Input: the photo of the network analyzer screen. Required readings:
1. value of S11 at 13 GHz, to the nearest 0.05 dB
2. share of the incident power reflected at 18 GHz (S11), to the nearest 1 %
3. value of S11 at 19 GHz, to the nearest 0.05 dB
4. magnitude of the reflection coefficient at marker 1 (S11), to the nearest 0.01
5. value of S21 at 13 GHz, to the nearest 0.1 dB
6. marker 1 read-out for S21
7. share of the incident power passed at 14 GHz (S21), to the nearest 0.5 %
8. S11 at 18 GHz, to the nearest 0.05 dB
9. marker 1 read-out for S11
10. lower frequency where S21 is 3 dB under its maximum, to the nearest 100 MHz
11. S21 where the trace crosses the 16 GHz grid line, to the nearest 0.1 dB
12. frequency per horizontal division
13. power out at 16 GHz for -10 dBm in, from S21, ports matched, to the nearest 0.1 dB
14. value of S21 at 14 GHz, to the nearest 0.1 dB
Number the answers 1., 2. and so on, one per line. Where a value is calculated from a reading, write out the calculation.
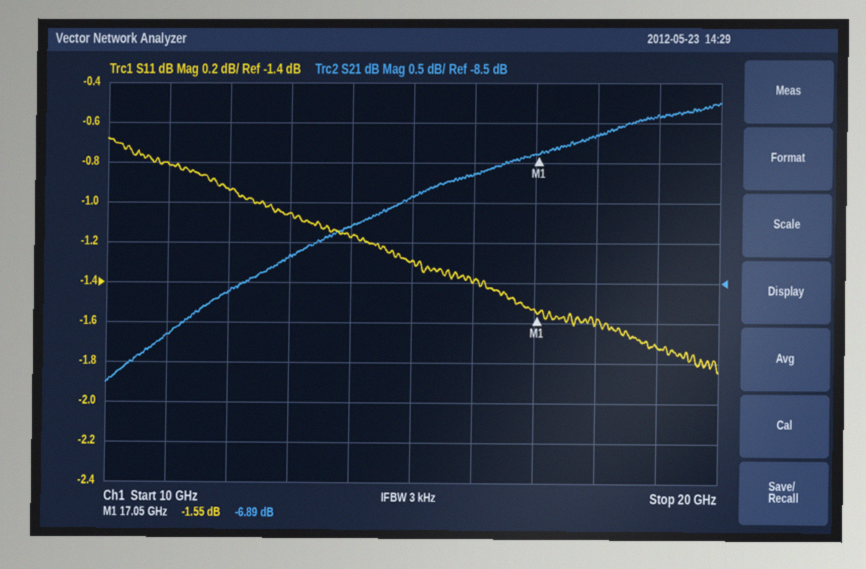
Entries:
1. -1.05 dB
2. 10^(-1.6/10) ≈ 69 %
3. -1.70 dB
4. 10^(-1.55/20) ≈ 0.84
5. -8.2 dB
6. -6.89 dB
7. 10^(-7.8/10) ≈ 16.6 %, so 16.5 % to the nearest 0.5 %
8. -1.60 dB
9. -1.55 dB
10. 10.8 GHz
11. -7.1 dB
12. 1 GHz
13. -10 dBm + (-7.1 dB) = -17.1 dBm
14. -7.8 dB
